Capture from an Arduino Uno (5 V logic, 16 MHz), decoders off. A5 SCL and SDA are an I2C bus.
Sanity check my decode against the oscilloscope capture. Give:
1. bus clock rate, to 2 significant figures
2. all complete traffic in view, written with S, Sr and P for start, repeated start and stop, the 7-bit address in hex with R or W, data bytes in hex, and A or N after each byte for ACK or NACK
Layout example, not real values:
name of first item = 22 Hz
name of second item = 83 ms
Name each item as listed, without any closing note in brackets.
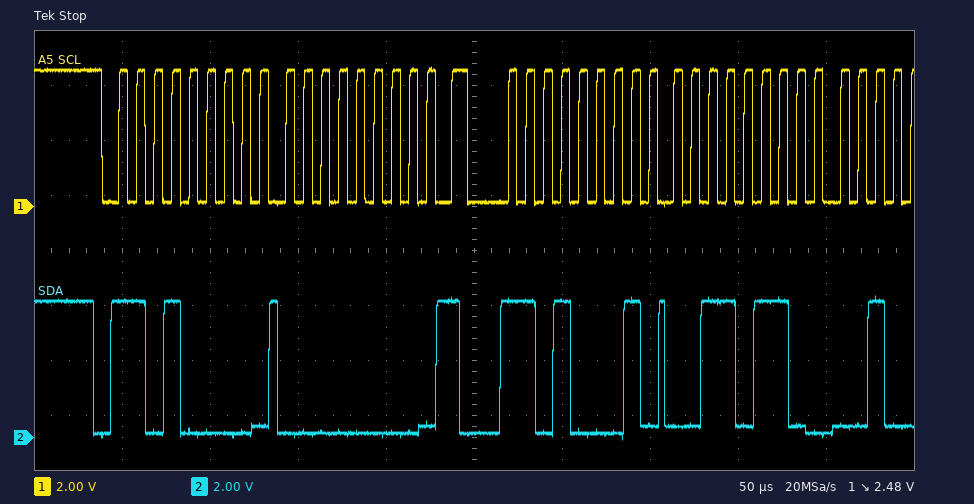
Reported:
bus clock rate, to 2 significant figures = 100 kHz
all complete traffic in view, written with S, Sr and P for start, repeated start and stop, the 7-bit address in hex with R or W, data bytes in hex, and A or N after each byte for ACK or NACK = S 68W A 00 A Sr 68R A 36 A
